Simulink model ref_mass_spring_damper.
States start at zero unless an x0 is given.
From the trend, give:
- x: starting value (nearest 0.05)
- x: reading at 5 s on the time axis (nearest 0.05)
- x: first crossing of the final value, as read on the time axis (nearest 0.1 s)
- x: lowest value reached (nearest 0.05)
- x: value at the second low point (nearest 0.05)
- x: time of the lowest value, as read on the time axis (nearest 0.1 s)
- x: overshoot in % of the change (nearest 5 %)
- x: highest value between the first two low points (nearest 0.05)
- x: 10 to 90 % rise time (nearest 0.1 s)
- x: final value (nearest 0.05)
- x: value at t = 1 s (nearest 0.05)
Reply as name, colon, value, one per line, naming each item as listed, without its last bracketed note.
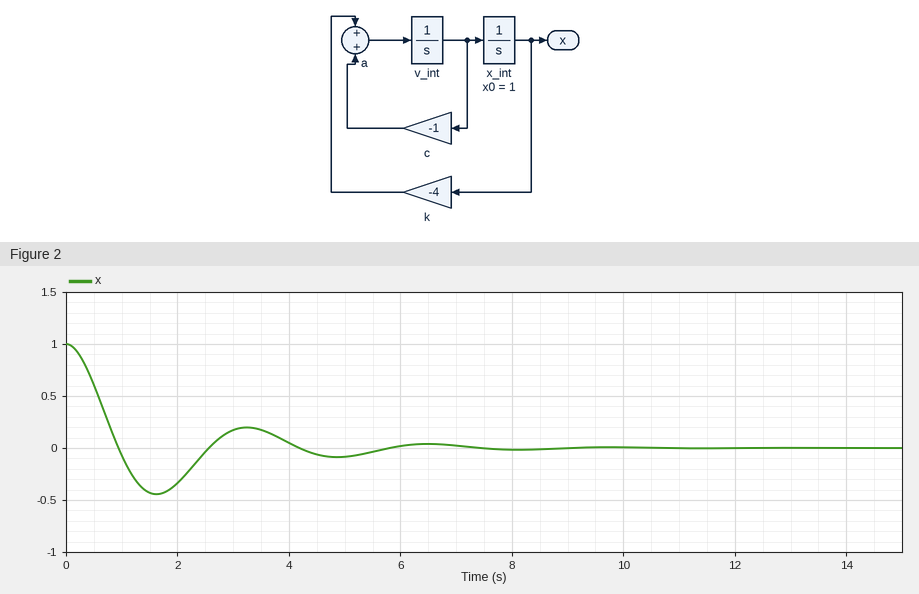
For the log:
x: starting value: 1.00
x: reading at 5 s on the time axis: -0.10
x: first crossing of the final value, as read on the time axis: 0.9 s
x: lowest value reached: -0.45
x: value at the second low point: -0.10
x: time of the lowest value, as read on the time axis: 1.6 s
x: overshoot in % of the change: 45 %
x: highest value between the first two low points: 0.20
x: 10 to 90 % rise time: 0.6 s
x: final value: 0.00
x: value at t = 1 s: -0.05
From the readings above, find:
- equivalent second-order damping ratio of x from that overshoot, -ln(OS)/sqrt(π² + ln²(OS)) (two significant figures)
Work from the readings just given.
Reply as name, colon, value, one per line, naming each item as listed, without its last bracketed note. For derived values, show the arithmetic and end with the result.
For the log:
equivalent second-order damping ratio of x from that overshoot, -ln(OS)/sqrt(π² + ln²(OS)): ln(0.45) = -0.799; 0.799 / sqrt(9.870 + 0.638) = 0.25
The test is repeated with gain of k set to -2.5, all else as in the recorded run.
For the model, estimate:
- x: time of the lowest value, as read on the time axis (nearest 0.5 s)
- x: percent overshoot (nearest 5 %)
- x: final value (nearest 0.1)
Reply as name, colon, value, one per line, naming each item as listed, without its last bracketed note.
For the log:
x: time of the lowest value, as read on the time axis: 2.0 s
x: percent overshoot: 35 %
x: final value: 0.0
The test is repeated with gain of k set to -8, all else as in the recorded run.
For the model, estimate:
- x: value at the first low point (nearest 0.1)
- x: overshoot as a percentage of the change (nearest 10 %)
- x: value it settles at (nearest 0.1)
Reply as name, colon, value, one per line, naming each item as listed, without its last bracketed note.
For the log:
x: value at the first low point: -0.6
x: overshoot as a percentage of the change: 60 %
x: value it settles at: 0.0
